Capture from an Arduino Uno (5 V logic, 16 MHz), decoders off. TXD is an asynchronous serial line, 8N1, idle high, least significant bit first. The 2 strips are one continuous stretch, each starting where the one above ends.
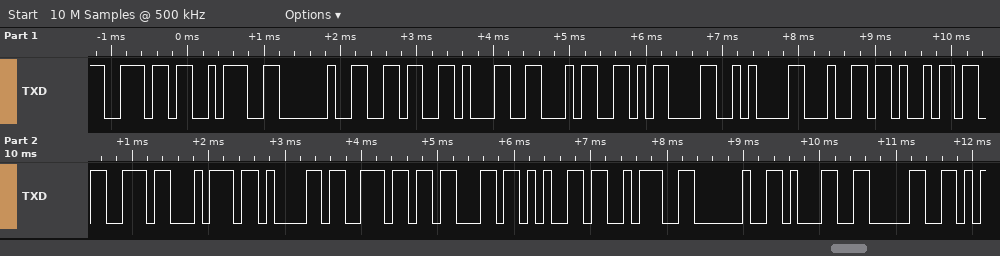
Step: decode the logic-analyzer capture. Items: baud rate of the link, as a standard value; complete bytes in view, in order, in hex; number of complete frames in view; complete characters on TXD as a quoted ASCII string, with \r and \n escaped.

9600 baud
6E 3A 20 36 31 34 0D 0A 64 69 73 74 61 6E 63 65 3A 20 31 30
20
"n: 614\r\ndistance: 10"
